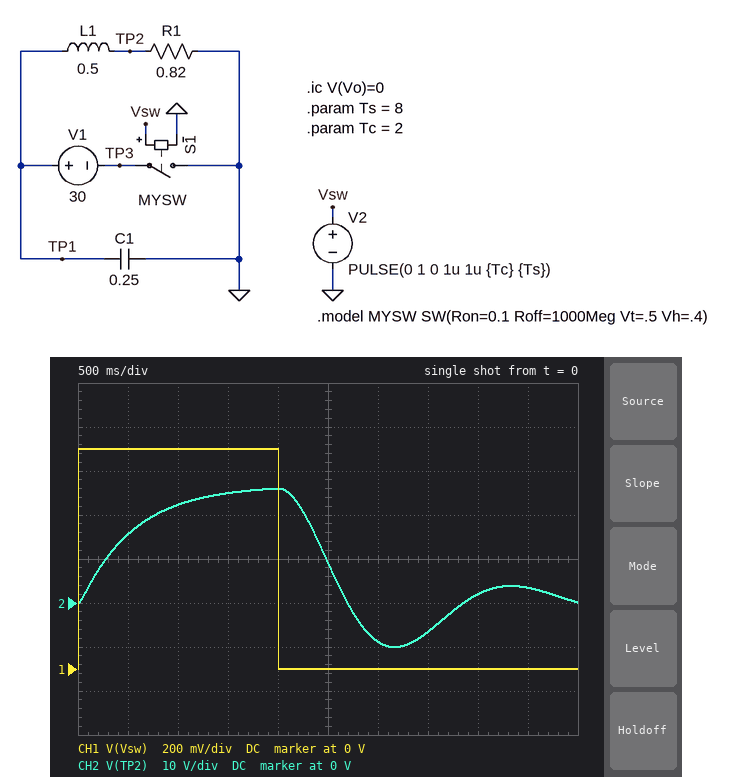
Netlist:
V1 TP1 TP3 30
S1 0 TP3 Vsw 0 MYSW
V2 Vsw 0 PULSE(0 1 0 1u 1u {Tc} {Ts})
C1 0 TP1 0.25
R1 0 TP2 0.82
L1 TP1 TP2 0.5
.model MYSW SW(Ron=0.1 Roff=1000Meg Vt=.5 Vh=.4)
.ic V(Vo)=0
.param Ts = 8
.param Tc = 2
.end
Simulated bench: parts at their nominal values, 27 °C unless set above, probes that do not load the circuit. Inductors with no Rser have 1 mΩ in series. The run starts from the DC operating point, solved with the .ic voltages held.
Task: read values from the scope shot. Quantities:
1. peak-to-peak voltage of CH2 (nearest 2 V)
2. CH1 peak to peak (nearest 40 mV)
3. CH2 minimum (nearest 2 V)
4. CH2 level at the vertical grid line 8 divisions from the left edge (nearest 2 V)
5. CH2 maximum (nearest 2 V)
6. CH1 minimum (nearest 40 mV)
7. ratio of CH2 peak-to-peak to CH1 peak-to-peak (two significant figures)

36 V
1.00 V
-10 V
2 V
26 V
0 V
36
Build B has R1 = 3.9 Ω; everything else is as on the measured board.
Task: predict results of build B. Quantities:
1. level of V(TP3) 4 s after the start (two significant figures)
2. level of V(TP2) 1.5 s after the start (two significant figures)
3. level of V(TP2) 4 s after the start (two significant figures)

-27 V
29 V
3.2 V
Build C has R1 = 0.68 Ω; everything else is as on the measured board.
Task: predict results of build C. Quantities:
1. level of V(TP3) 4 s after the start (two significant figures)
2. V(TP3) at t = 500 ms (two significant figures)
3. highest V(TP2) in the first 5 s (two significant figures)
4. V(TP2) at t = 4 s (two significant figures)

-17 V
-1.9 V
25 V
3.2 V
